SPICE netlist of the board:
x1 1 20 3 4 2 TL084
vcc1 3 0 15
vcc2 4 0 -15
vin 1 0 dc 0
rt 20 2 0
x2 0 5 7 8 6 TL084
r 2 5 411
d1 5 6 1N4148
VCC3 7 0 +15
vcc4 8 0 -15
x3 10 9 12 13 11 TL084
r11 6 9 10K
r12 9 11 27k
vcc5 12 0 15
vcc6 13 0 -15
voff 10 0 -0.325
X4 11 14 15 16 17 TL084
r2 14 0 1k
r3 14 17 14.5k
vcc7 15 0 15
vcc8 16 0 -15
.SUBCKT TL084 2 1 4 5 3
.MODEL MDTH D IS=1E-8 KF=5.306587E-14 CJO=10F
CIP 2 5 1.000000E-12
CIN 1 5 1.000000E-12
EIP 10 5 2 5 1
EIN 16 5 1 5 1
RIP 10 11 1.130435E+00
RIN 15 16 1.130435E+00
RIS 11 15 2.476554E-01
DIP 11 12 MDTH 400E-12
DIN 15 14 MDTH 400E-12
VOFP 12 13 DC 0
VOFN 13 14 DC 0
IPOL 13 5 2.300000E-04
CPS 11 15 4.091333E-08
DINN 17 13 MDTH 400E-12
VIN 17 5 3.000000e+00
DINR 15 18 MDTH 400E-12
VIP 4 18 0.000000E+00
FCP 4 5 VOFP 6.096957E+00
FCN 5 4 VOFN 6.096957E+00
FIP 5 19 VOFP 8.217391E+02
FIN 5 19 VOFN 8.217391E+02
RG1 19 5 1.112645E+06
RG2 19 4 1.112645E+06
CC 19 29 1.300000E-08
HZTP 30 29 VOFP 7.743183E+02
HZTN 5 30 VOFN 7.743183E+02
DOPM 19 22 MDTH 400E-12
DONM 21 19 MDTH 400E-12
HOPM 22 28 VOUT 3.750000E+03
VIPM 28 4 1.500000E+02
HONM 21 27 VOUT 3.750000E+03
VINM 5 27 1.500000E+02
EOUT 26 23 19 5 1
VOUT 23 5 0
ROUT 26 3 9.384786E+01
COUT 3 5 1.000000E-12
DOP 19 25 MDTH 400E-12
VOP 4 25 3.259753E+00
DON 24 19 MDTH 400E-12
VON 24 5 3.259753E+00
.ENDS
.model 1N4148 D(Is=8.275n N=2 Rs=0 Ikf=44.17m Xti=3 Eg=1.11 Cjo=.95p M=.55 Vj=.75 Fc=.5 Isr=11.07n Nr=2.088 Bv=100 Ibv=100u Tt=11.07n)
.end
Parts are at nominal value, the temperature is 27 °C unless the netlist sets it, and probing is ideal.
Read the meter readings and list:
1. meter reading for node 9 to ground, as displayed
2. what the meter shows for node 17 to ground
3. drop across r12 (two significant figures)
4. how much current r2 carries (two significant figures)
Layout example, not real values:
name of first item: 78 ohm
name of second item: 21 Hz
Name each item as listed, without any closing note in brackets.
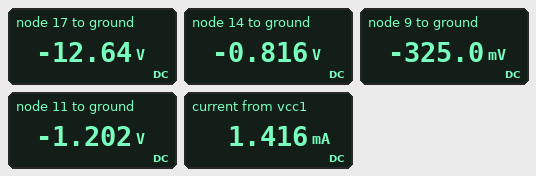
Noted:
meter reading for node 9 to ground, as displayed: -325.0 mV
what the meter shows for node 17 to ground: -12.64 V
drop across r12: 880 mV
how much current r2 carries: 820 µA
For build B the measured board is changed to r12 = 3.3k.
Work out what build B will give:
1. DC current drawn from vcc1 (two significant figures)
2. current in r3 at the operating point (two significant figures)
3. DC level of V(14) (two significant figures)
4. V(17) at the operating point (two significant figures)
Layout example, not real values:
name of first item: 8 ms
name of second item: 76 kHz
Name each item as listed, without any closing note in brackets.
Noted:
DC current drawn from vcc1: 1.4 mA
current in r3 at the operating point: 430 µA
DC level of V(14): -430 mV
V(17) at the operating point: -6.7 V
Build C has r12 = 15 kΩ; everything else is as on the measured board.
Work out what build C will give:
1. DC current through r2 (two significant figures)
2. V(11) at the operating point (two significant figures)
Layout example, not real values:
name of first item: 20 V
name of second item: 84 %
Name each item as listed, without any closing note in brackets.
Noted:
DC current through r2: 810 µA
V(11) at the operating point: -810 mV
